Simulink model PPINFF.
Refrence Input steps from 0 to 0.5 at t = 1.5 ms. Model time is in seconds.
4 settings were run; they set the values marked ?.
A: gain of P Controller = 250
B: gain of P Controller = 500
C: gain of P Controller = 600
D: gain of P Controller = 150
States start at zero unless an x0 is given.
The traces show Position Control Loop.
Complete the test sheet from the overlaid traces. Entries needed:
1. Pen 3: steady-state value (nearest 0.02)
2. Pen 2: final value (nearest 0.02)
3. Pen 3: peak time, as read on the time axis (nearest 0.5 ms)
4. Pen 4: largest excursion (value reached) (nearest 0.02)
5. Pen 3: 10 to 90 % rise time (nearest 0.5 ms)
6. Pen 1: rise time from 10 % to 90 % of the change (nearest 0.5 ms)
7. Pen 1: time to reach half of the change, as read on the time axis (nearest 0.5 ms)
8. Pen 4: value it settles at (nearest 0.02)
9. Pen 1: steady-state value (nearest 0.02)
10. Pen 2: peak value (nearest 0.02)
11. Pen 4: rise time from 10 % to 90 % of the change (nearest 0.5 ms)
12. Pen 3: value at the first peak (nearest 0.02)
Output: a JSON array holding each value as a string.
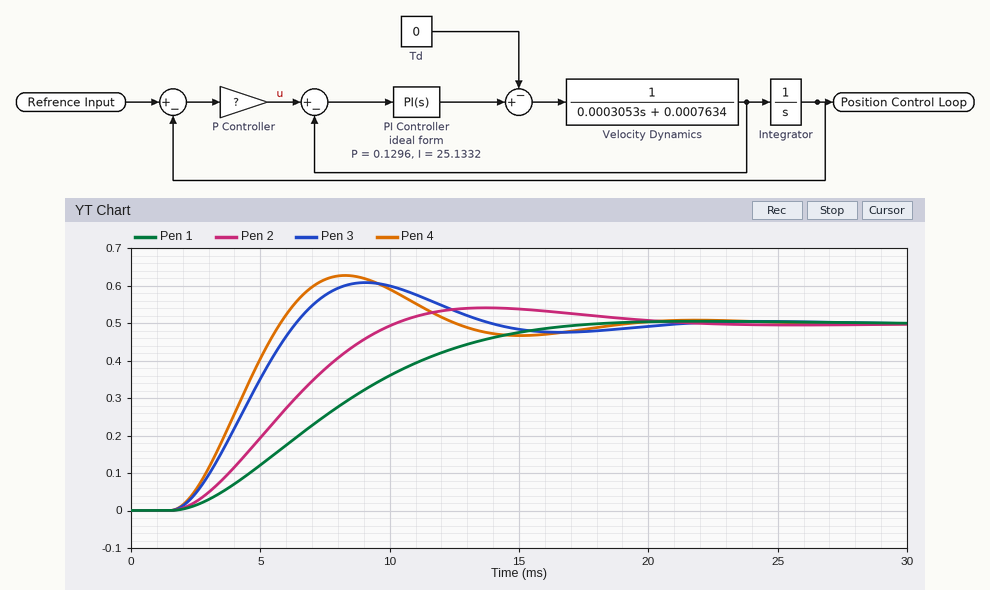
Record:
["0.50", "0.50", "9.0 ms", "0.62", "3.5 ms", "10.0 ms", "7.5 ms", "0.50", "0.50", "0.54", "3.0 ms", "0.60"]
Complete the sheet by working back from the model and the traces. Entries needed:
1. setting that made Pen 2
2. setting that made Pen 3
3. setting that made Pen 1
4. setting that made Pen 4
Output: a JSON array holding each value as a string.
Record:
["A", "B", "D", "C"]
